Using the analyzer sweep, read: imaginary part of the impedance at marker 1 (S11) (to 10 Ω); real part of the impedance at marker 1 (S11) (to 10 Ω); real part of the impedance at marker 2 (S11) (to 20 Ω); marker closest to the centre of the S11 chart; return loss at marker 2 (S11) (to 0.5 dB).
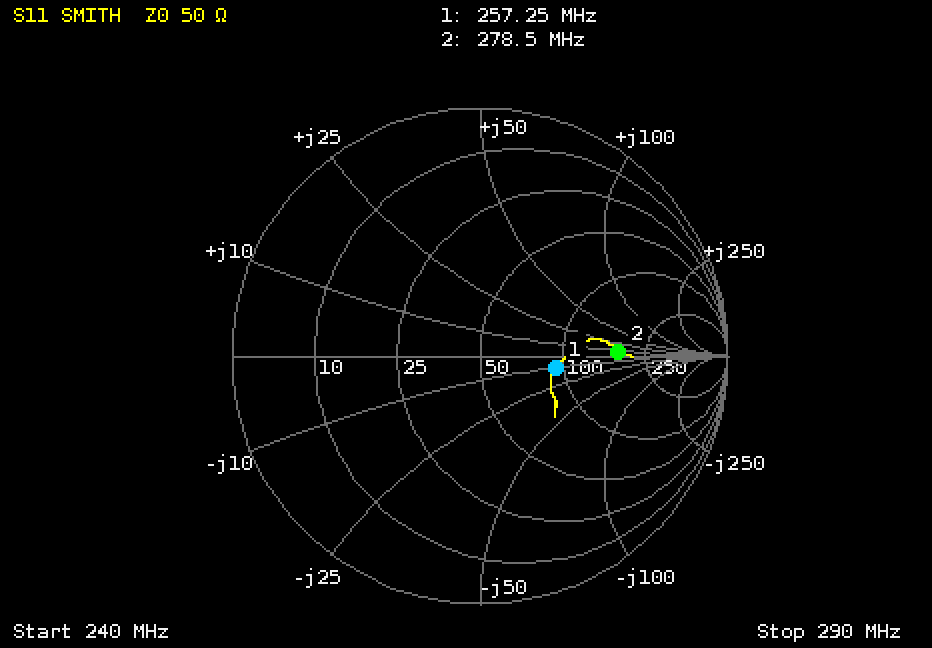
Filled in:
-10 Ω
90 Ω
180 Ω
marker 1
5.0 dB
